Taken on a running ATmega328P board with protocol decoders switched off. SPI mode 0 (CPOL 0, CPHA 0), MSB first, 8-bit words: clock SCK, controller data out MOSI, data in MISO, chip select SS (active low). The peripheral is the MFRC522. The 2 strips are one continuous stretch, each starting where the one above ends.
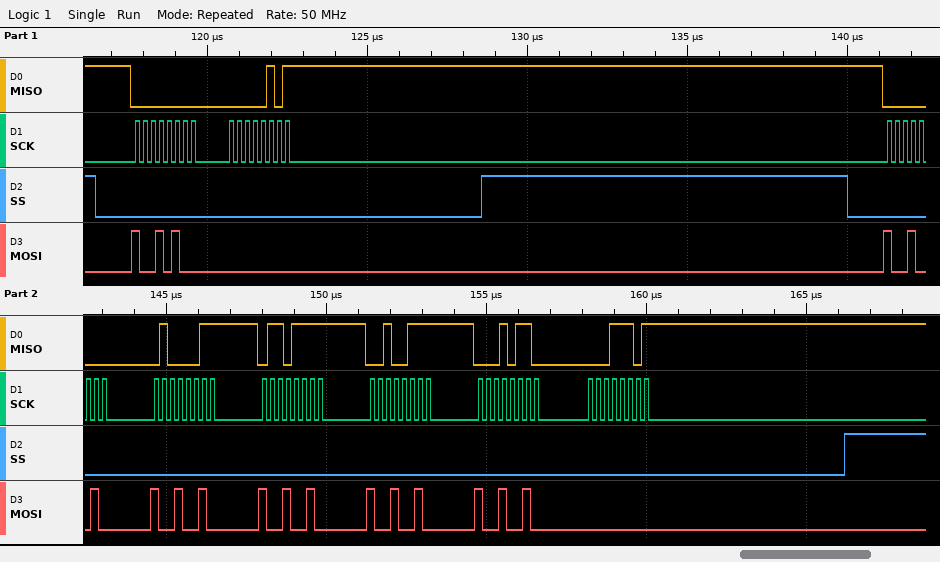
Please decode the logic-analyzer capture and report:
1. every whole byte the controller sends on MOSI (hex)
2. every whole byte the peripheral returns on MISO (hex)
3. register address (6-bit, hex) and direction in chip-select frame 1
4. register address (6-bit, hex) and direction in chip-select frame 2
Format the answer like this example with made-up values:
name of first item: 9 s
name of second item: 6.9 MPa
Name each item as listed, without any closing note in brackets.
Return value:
every whole byte the controller sends on MOSI: 94 00 92 92 92 92 92 00
every whole byte the peripheral returns on MISO: 00 05 00 43 6F 27 16 1D
register address (6-bit, hex) and direction in chip-select frame 1: 0x0A read
register address (6-bit, hex) and direction in chip-select frame 2: 0x09 read
